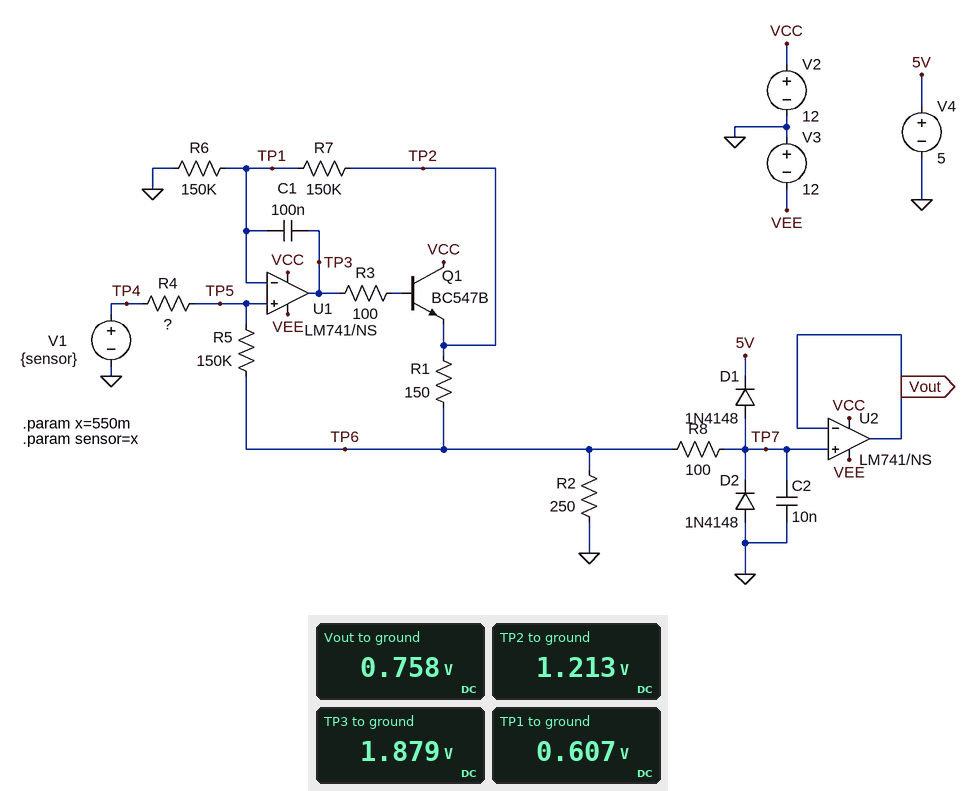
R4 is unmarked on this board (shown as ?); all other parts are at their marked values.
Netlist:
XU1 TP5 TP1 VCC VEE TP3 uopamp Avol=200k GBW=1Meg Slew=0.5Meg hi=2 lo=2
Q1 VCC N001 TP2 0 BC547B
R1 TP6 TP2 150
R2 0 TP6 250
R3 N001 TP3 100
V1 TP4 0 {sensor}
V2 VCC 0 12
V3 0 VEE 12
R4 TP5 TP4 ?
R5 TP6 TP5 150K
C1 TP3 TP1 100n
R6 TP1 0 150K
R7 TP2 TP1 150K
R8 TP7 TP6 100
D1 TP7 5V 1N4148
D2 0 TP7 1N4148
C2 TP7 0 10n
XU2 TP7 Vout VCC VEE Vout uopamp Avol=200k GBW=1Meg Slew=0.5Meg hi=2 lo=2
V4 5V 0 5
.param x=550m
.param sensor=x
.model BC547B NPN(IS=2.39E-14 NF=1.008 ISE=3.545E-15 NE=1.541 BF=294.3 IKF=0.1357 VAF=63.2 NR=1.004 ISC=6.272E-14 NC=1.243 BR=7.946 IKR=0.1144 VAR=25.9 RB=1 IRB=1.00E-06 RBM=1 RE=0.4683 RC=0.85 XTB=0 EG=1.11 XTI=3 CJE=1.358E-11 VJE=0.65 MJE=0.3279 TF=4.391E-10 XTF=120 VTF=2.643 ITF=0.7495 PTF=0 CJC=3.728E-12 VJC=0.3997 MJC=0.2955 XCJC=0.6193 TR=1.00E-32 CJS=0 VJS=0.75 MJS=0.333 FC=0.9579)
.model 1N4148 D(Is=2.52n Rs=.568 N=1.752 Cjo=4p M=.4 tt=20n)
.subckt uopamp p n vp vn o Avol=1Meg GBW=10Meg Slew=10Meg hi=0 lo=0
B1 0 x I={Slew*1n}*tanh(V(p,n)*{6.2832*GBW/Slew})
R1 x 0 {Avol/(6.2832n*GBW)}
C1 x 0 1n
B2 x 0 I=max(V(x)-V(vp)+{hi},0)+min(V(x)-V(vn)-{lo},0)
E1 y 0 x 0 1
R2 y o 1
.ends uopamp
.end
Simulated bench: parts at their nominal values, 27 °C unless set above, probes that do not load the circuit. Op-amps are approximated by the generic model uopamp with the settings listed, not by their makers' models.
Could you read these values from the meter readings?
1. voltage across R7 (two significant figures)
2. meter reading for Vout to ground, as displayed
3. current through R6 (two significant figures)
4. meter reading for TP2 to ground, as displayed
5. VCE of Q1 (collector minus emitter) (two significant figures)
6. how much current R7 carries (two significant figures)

610 mV
0.758 V
4.0 µA
1.213 V
11 V
4.0 µA
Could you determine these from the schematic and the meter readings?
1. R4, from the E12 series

56 kΩ
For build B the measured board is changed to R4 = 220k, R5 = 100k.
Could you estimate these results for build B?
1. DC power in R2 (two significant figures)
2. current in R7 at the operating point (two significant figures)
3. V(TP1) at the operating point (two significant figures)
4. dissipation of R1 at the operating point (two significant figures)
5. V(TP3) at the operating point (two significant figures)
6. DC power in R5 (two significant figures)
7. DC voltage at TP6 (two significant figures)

9.3 mW
8.1 µA
1.2 V
5.6 mW
3.1 V
930 nW
1.5 V
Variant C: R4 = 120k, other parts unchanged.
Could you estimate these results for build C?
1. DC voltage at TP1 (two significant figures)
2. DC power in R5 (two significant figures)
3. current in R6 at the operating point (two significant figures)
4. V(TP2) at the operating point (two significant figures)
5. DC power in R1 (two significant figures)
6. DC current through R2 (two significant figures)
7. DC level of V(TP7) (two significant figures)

690 mV
200 nW
4.6 µA
1.4 V
1.8 mW
3.4 mA
860 mV
